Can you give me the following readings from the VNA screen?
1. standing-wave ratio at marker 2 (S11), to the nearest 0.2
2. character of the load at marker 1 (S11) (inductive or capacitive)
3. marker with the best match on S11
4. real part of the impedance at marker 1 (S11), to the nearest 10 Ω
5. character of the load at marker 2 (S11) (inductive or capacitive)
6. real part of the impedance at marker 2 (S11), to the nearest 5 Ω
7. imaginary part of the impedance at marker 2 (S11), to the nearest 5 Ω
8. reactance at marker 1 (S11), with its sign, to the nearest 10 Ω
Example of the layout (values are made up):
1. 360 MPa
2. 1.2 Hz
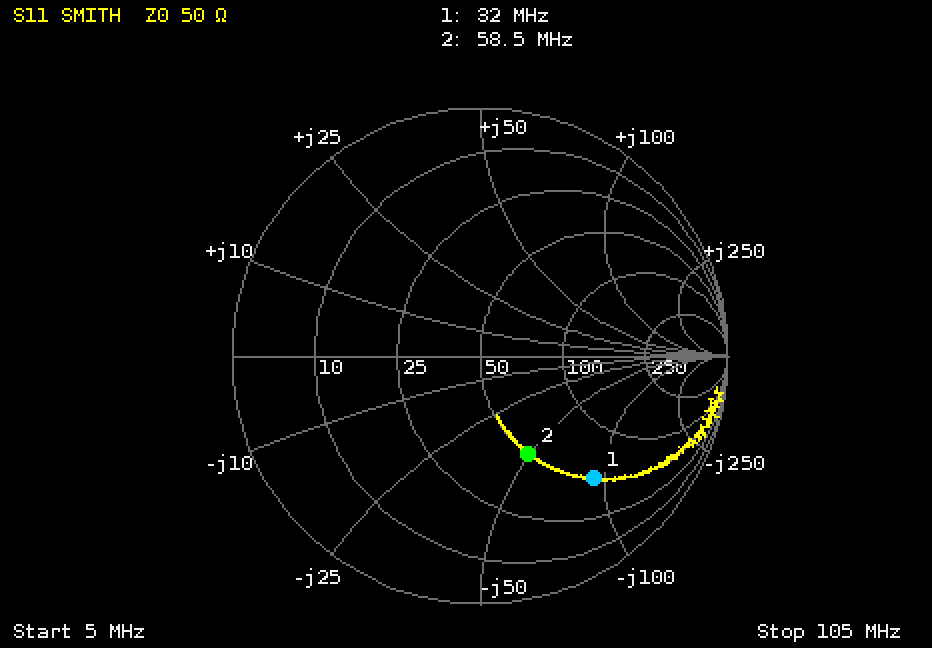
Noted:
1. 2.6
2. capacitive
3. marker 2
4. 50 Ω
5. capacitive
6. 50 Ω
7. -50 Ω
8. -90 Ω
